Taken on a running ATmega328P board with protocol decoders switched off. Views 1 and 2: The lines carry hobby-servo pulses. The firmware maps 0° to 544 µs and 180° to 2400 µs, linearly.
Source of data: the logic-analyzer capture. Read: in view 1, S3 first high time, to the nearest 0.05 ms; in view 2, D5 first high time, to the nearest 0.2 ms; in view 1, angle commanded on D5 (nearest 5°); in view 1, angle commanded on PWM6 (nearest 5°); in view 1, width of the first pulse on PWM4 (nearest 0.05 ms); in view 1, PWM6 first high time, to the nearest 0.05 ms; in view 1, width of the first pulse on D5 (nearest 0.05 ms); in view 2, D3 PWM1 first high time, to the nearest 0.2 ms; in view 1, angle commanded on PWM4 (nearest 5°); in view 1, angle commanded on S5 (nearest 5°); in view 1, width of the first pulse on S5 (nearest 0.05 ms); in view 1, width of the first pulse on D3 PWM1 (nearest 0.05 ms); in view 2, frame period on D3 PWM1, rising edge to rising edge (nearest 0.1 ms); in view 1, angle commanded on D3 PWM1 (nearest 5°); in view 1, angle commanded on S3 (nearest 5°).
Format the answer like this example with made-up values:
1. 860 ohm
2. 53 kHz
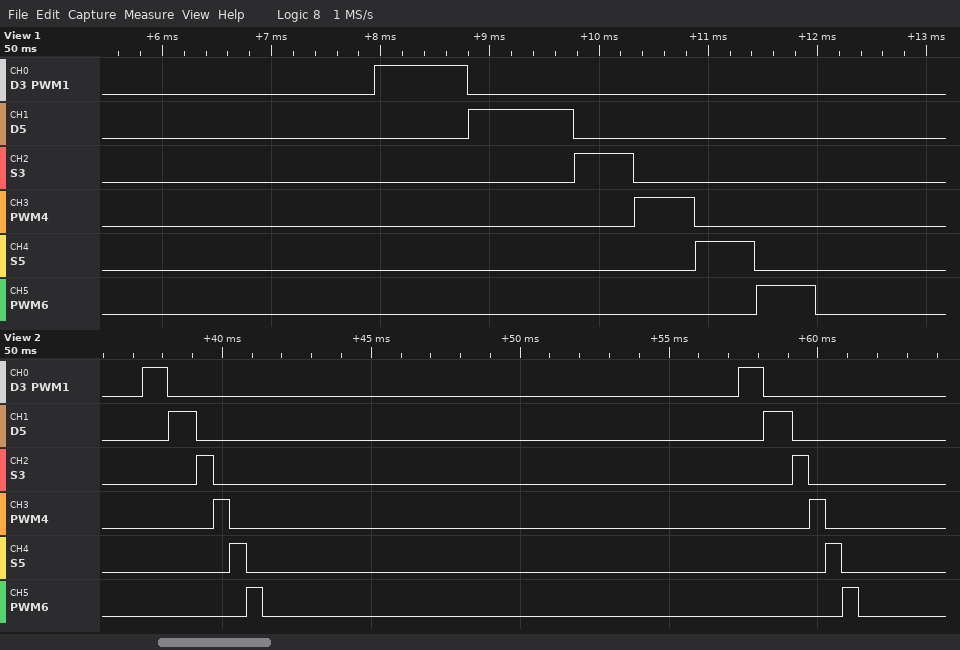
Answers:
1. 0.55 ms
2. 1.0 ms
3. 40°
4. 0°
5. 0.55 ms
6. 0.55 ms
7. 0.95 ms
8. 0.8 ms
9. 0°
10. 0°
11. 0.55 ms
12. 0.85 ms
13. 20.0 ms
14. 30°
15. 0°
